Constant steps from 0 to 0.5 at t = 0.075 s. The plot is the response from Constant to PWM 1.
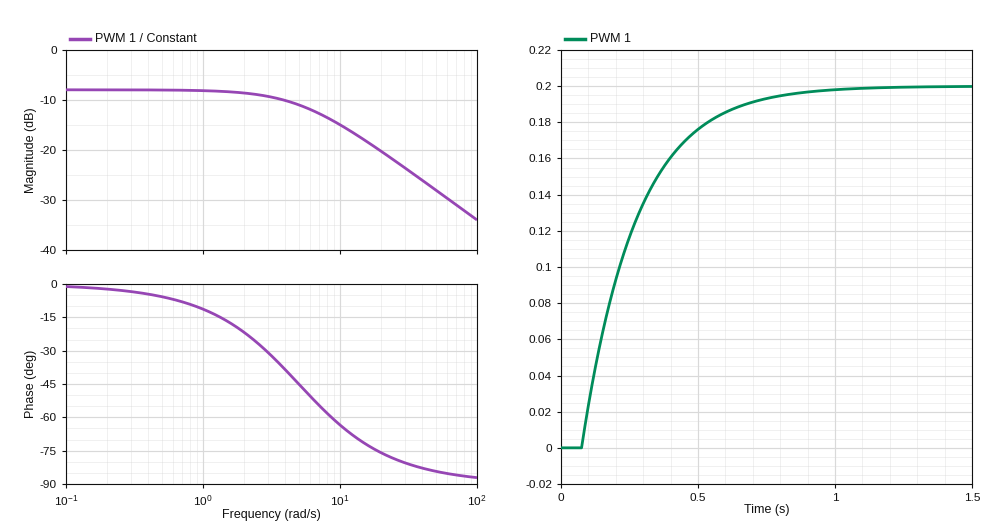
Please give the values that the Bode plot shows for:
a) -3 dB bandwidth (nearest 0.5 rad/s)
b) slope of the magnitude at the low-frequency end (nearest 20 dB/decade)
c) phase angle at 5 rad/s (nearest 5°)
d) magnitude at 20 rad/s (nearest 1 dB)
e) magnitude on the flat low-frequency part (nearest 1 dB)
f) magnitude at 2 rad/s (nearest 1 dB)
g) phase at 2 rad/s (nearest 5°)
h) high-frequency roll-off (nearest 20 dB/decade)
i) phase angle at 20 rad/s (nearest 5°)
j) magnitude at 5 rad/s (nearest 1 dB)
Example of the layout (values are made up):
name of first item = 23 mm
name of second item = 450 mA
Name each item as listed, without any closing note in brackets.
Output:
-3 dB bandwidth = 5.0 rad/s
slope of the magnitude at the low-frequency end = 0 dB/decade
phase angle at 5 rad/s = -45°
magnitude at 20 rad/s = -20 dB
magnitude on the flat low-frequency part = -8 dB
magnitude at 2 rad/s = -9 dB
phase at 2 rad/s = -20°
high-frequency roll-off = -20 dB/decade
phase angle at 20 rad/s = -75°
magnitude at 5 rad/s = -11 dB
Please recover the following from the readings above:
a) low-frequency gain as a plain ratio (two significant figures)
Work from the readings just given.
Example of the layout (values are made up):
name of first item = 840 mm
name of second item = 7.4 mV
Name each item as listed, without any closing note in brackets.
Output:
low-frequency gain as a plain ratio = 0.40
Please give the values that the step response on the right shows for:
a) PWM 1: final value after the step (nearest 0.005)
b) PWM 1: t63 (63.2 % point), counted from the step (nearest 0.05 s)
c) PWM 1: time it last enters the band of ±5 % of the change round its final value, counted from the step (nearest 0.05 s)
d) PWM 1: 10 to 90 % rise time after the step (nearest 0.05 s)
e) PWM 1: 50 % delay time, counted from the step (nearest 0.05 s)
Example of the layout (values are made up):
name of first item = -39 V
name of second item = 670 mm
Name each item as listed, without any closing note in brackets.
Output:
PWM 1: final value after the step = 0.200
PWM 1: t63 (63.2 % point), counted from the step = 0.20 s
PWM 1: time it last enters the band of ±5 % of the change round its final value, counted from the step = 0.60 s
PWM 1: 10 to 90 % rise time after the step = 0.45 s
PWM 1: 50 % delay time, counted from the step = 0.15 s
